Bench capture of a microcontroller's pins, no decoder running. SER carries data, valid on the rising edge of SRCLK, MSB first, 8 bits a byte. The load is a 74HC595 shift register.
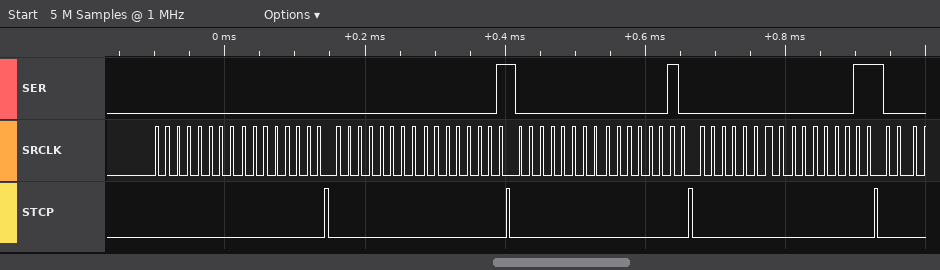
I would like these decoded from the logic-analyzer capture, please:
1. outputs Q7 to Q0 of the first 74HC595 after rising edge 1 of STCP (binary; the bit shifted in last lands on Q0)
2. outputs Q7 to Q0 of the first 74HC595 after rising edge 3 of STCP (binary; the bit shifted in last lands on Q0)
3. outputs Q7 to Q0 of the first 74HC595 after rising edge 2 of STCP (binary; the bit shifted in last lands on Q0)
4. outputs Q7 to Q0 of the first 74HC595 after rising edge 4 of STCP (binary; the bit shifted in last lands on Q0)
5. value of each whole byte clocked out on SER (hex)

00000000
00000010
00000001
00000011
0x00 0x00 0x00 0x01 0x00 0x02 0x00 0x03
